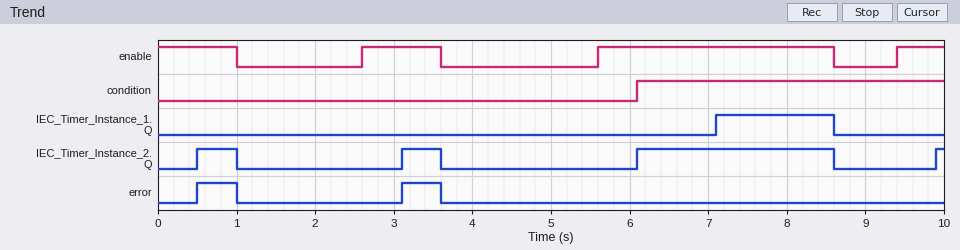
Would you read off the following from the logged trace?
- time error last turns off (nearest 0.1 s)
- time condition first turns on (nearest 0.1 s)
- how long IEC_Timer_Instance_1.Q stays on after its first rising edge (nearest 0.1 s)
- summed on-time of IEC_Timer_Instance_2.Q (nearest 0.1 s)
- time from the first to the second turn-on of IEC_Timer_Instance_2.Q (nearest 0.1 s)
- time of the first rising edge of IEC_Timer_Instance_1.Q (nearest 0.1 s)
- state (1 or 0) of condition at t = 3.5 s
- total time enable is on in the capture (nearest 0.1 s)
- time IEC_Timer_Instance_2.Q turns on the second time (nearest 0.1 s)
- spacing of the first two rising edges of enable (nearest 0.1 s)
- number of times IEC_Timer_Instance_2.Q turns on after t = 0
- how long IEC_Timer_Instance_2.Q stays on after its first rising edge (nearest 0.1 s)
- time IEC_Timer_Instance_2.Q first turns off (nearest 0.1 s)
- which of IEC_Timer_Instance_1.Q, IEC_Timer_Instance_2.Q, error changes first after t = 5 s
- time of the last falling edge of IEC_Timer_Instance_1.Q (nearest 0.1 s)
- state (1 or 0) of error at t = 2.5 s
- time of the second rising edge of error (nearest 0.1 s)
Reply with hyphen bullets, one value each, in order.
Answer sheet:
- 3.6 s
- 6.1 s
- 1.5 s
- 3.6 s
- 2.6 s
- 7.1 s
- 0
- 5.6 s
- 3.1 s
- 3.0 s
- 4
- 0.5 s
- 1.0 s
- IEC_Timer_Instance_2.Q
- 8.6 s
- 0
- 3.1 s
